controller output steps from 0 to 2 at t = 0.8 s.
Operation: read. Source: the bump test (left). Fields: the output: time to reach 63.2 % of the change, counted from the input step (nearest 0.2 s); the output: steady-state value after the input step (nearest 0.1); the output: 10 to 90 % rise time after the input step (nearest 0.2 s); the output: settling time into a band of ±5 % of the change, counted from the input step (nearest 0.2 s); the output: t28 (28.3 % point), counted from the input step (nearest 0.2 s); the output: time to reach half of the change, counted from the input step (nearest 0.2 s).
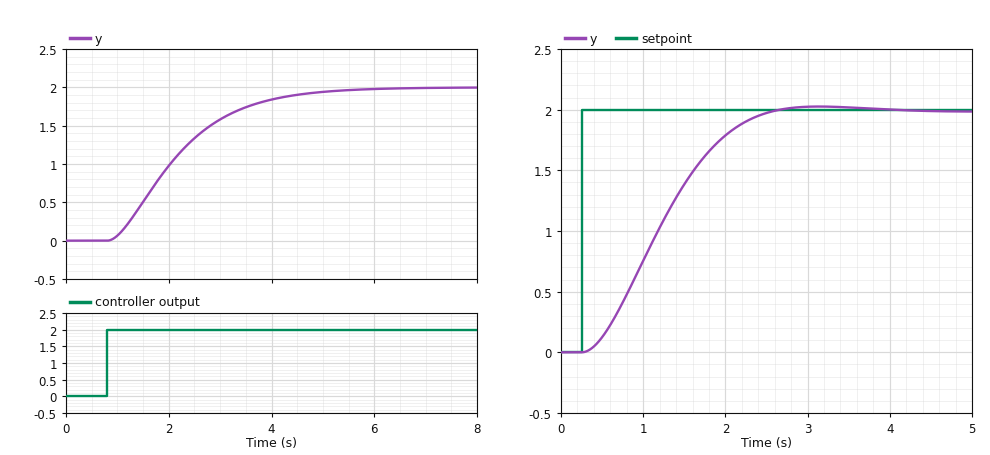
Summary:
1.6 s
2.0
2.6 s
3.6 s
0.8 s
1.2 s
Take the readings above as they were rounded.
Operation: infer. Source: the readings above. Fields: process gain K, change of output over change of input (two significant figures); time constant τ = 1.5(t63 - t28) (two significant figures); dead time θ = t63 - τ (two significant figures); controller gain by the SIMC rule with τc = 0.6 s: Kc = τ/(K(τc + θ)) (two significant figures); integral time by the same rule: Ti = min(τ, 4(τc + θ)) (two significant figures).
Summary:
1.0
1.2 s
0.40 s
1.2
1.2 s
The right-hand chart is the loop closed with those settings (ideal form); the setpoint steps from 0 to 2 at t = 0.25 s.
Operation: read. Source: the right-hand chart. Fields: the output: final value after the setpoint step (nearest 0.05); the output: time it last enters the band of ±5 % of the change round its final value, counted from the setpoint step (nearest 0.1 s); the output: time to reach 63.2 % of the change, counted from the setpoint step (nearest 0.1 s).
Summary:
2.00
2.0 s
1.1 s
